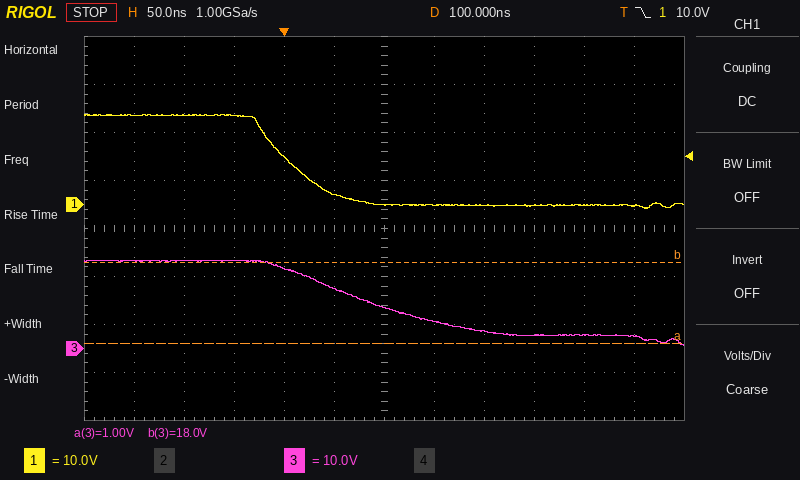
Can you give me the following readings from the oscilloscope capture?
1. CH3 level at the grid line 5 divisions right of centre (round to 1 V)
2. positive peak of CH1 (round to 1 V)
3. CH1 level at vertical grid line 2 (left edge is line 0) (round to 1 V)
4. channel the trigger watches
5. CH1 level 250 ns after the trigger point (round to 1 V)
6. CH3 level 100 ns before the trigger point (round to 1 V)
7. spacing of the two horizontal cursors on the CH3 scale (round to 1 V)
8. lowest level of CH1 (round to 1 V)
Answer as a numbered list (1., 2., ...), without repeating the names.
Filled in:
1. 3 V
2. 19 V
3. 19 V
4. CH1
5. 0 V
6. 18 V
7. 17 V
8. -1 V
